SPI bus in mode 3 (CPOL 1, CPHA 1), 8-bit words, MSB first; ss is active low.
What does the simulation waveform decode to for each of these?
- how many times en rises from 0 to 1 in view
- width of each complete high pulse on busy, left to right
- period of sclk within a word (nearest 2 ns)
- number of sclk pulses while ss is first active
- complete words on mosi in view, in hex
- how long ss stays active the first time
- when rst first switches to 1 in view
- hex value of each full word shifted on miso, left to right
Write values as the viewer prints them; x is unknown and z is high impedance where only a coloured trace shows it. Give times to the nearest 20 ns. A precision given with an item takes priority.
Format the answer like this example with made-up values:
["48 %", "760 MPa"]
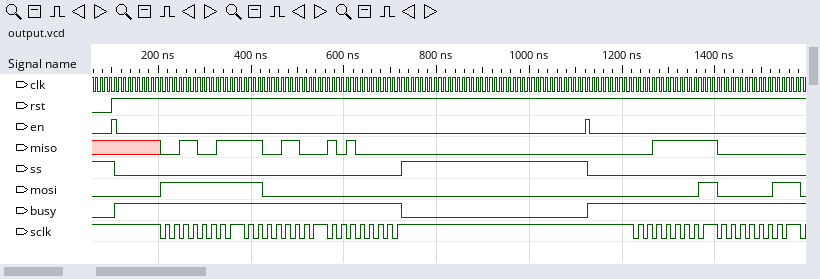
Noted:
["2", "620 ns", "20 ns", "24", "FF, C0, 00, 01, 03", "620 ns", "100 ns", "33, CC, A0, 3F, 00"]
